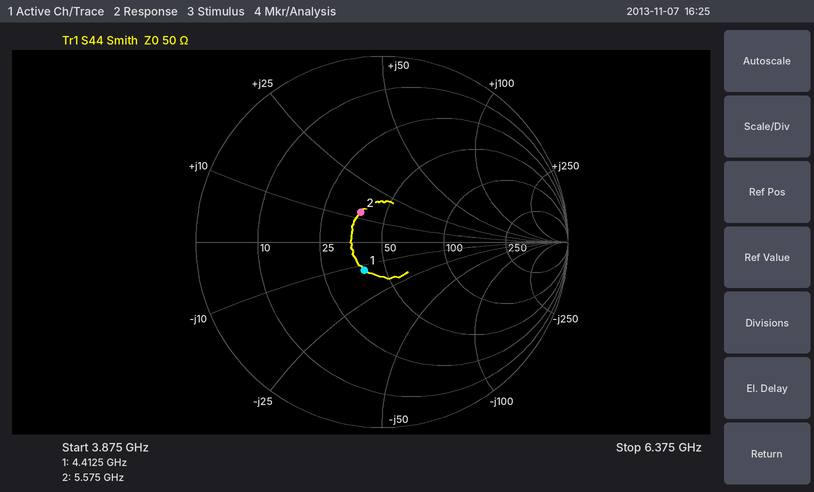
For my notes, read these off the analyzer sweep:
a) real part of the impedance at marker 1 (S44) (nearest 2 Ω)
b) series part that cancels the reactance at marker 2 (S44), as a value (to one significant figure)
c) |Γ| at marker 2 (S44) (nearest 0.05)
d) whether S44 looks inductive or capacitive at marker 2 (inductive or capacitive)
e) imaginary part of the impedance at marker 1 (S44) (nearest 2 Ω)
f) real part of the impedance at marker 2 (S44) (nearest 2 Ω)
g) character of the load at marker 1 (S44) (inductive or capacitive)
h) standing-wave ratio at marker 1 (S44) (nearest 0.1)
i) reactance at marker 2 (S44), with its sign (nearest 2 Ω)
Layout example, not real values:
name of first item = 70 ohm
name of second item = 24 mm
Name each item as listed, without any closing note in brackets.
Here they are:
real part of the impedance at marker 1 (S44) = 40 Ω
series part that cancels the reactance at marker 2 (S44), as a value = 2 pF
|Γ| at marker 2 (S44) = 0.20
whether S44 looks inductive or capacitive at marker 2 = inductive
imaginary part of the impedance at marker 1 (S44) = -12 Ω
real part of the impedance at marker 2 (S44) = 38 Ω
character of the load at marker 1 (S44) = capacitive
standing-wave ratio at marker 1 (S44) = 1.4
reactance at marker 2 (S44), with its sign = +12 Ω
